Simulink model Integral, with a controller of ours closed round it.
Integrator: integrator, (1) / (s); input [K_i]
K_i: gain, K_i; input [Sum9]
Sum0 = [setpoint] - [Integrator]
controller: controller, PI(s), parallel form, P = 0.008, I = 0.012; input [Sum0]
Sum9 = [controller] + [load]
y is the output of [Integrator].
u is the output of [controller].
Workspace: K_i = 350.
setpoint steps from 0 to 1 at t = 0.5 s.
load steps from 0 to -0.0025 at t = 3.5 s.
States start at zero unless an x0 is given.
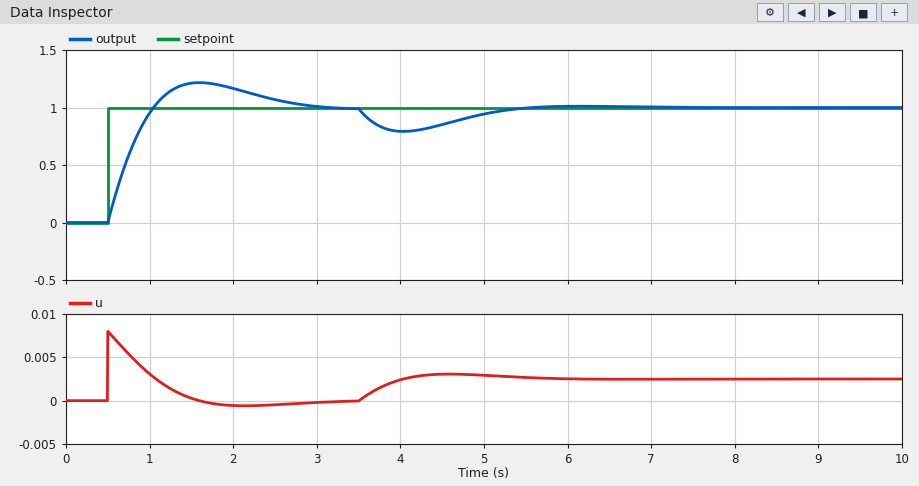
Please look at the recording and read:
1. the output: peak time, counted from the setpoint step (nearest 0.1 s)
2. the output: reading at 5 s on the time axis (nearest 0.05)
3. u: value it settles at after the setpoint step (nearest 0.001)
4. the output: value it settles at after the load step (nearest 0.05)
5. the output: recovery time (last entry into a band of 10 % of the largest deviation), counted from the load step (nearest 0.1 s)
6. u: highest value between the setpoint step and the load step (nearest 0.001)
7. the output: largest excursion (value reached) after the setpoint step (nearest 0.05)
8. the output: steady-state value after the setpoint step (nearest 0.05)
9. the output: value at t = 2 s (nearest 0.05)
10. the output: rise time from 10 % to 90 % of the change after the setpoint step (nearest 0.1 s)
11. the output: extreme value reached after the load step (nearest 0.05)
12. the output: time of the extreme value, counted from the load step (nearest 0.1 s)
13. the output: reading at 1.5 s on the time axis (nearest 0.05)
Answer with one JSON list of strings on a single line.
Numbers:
["1.1 s", "0.95", "0.000", "1.00", "1.8 s", "0.008", "1.20", "1.00", "1.15", "0.4 s", "0.80", "0.5 s", "1.20"]
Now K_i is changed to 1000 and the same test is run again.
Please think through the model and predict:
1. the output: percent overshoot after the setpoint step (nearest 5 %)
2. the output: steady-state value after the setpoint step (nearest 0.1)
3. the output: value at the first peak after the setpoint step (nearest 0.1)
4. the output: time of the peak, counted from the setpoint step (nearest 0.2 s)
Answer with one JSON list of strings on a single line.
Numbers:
["10 %", "1.0", "1.1", "0.6 s"]
